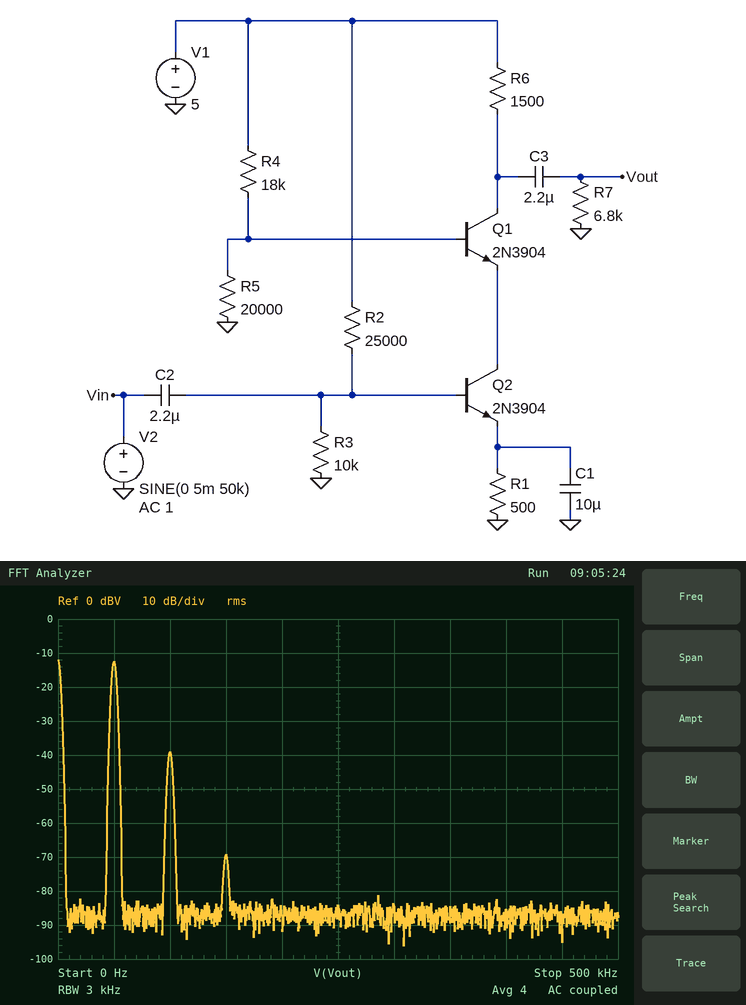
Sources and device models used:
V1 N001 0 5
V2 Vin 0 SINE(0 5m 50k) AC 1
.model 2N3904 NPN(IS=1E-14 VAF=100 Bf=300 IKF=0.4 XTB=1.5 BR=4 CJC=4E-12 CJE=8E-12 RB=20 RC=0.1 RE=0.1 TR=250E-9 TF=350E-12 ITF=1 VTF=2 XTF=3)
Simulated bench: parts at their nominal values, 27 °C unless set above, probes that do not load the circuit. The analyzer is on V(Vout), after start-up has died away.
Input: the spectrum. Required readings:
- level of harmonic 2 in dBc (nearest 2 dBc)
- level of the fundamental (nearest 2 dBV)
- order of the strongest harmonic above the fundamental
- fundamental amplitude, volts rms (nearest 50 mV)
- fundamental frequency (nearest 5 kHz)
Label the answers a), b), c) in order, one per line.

a) -26 dBc
b) -12 dBV
c) 2
d) 250 mV
e) 50 kHz
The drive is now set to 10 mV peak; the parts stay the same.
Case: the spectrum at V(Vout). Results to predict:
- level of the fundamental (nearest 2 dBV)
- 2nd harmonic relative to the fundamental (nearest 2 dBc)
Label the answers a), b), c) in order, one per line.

a) -6 dBV
b) -20 dBc
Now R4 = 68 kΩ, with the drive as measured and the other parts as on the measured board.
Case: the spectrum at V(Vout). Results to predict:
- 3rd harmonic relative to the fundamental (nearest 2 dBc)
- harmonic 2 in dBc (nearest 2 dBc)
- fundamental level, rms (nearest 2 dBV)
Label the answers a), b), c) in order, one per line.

a) -52 dBc
b) -30 dBc
c) -24 dBV
